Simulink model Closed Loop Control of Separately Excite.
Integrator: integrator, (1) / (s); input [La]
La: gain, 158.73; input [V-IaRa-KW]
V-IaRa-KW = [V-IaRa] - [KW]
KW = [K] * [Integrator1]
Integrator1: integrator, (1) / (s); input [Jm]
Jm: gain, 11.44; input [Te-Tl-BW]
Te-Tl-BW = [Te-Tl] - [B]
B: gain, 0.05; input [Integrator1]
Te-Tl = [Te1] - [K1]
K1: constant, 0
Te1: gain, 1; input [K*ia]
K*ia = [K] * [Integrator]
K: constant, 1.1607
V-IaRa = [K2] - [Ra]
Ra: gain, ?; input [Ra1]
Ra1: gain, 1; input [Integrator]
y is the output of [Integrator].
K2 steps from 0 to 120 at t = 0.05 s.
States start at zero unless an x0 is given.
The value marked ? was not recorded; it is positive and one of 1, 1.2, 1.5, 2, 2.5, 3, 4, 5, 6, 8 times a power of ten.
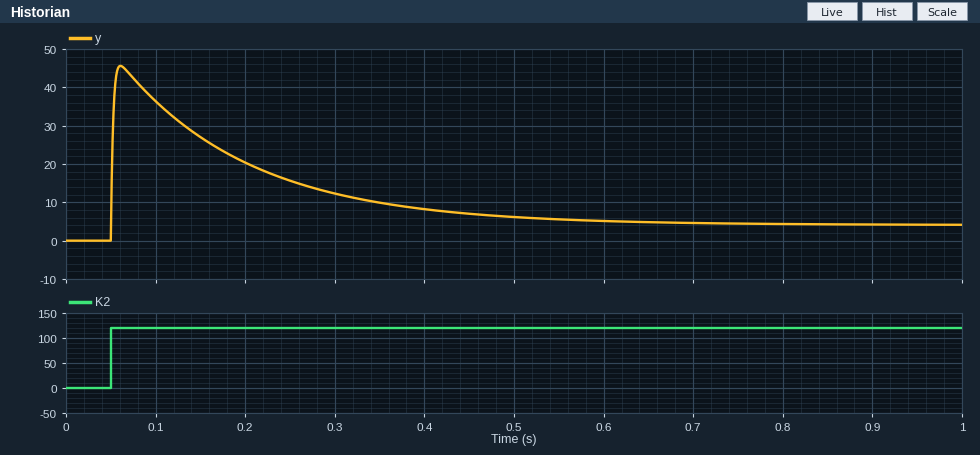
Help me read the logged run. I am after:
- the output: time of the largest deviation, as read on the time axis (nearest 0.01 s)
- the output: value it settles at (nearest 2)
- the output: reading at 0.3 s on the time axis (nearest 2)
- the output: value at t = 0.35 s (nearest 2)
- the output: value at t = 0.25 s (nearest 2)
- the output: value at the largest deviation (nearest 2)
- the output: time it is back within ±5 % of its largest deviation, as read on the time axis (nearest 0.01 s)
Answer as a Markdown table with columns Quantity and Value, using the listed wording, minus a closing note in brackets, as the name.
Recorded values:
| Quantity | Value |
|---|---|
| the output: time of the largest deviation, as read on the time axis | 0.06 s |
| the output: value it settles at | 4 |
| the output: reading at 0.3 s on the time axis | 12 |
| the output: value at t = 0.35 s | 10 |
| the output: value at t = 0.25 s | 16 |
| the output: value at the largest deviation | 46 |
| the output: time it is back within ±5 % of its largest deviation, as read on the time axis | 0.49 s |
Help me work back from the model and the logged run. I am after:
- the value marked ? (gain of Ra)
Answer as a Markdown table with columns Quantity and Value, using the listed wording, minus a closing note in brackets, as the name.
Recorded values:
| Quantity | Value |
|---|---|
| the value marked ? | 2.5 |
